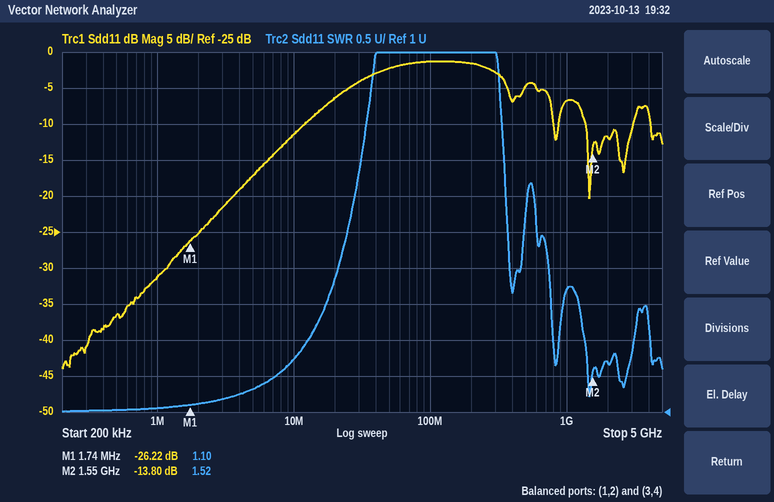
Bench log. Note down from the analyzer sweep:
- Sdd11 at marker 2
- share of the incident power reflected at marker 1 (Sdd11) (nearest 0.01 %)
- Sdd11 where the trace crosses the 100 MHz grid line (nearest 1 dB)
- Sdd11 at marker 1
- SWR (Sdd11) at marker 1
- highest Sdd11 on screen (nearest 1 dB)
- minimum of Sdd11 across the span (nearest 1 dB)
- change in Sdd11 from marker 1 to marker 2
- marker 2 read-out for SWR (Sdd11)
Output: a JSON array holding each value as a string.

["-13.80 dB", "0.24 %", "-1 dB", "-26.22 dB", "1.10", "-1 dB", "-44 dB", "12.42 dB", "1.52"]
